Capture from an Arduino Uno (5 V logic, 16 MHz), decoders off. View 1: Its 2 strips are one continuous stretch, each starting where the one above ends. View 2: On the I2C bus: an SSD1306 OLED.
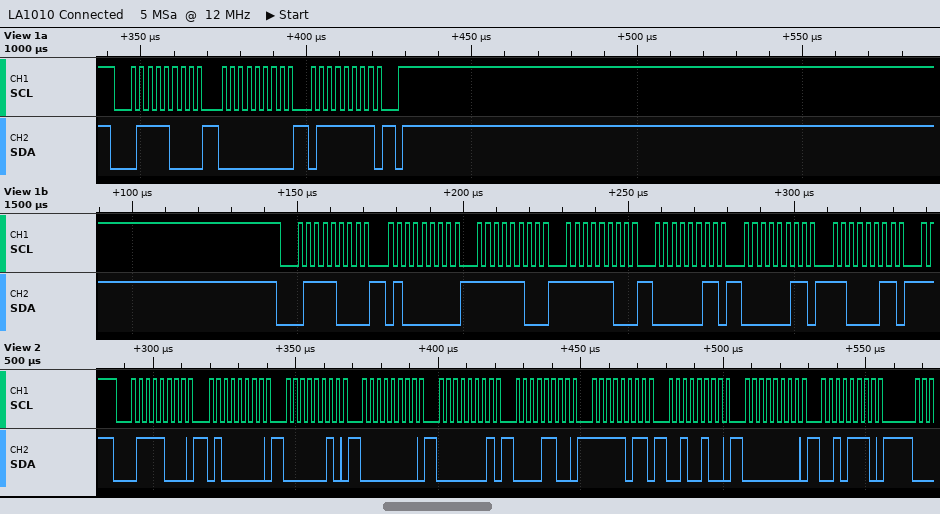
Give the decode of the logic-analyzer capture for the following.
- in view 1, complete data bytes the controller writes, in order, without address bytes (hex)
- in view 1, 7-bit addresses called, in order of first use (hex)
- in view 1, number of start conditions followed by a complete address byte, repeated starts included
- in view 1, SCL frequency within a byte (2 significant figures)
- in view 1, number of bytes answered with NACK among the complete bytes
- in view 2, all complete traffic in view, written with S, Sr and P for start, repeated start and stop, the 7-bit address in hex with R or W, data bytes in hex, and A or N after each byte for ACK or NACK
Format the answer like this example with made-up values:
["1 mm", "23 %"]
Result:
["00 7F 40 FC FC 03 03 C3", "0x3C", "2", "400 kHz", "0", "S 3CW A 40 A 02 A 00 A 01 A 0C A FB A 24 A 00 A 2E A"]
